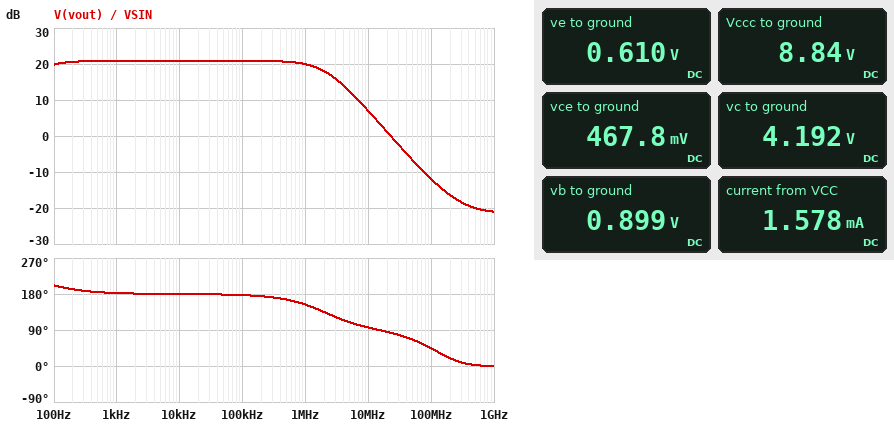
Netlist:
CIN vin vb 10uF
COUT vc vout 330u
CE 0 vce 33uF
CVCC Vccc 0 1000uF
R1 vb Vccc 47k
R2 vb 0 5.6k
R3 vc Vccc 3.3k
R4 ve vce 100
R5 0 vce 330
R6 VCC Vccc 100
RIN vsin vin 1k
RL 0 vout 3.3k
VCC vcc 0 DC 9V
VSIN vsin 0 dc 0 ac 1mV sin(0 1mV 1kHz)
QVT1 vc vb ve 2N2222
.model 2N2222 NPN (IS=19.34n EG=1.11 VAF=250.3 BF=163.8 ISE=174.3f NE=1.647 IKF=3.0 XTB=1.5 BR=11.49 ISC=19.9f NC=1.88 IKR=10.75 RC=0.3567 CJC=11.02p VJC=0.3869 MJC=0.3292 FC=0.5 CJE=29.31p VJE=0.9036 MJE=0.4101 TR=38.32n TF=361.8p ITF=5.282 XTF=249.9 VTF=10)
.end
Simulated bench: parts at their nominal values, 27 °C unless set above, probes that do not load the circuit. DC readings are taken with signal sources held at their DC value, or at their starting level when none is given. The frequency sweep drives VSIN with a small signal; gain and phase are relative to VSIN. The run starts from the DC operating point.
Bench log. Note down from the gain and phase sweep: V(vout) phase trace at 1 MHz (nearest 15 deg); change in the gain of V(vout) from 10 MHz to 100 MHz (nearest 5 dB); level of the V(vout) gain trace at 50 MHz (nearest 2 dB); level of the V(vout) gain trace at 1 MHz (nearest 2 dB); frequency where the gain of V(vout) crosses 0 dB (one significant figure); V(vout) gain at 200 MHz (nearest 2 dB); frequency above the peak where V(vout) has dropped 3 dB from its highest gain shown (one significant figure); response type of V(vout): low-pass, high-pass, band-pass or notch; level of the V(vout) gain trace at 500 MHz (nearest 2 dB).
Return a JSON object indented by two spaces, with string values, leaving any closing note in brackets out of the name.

{
  "V(vout) phase trace at 1 MHz": "150 deg",
  "change in the gain of V(vout) from 10 MHz to 100 MHz": "-20 dB",
  "level of the V(vout) gain trace at 50 MHz": "-6 dB",
  "level of the V(vout) gain trace at 1 MHz": "20 dB",
  "frequency where the gain of V(vout) crosses 0 dB": "20 MHz",
  "V(vout) gain at 200 MHz": "-16 dB",
  "frequency above the peak where V(vout) has dropped 3 dB from its highest gain shown": "2 MHz",
  "response type of V(vout): low-pass, high-pass, band-pass or notch": "low-pass",
  "level of the V(vout) gain trace at 500 MHz": "-20 dB"
}
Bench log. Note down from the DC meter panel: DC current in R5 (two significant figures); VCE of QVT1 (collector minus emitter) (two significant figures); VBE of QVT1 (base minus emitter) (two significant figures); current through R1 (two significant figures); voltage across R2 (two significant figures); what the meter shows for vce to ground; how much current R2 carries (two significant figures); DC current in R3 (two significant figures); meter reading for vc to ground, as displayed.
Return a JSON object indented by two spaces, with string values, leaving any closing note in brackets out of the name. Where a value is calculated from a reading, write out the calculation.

{
  "DC current in R5": "(467.8 mV) / 330 Ω = 1.4 mA",
  "VCE of QVT1 (collector minus emitter)": "4.192 V - 610 mV = 3.6 V",
  "VBE of QVT1 (base minus emitter)": "899 mV - 610 mV = 290 mV",
  "current through R1": "(8.84 V - 899 mV) / 47 kΩ = 170 µA",
  "voltage across R2": "899 mV = 900 mV",
  "what the meter shows for vce to ground": "467.8 mV",
  "how much current R2 carries": "(899 mV) / 5.6 kΩ = 160 µA",
  "DC current in R3": "(8.84 V - 4.192 V) / 3.3 kΩ = 1.4 mA",
  "meter reading for vc to ground, as displayed": "4.192 V"
}
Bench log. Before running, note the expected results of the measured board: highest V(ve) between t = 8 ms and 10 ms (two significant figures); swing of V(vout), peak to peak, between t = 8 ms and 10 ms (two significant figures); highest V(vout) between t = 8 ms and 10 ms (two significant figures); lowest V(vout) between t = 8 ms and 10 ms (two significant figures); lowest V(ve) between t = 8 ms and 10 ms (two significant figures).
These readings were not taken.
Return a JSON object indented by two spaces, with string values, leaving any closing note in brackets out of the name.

{
  "highest V(ve) between t = 8 ms and 10 ms": "610 mV",
  "swing of V(vout), peak to peak, between t = 8 ms and 10 ms": "22 mV",
  "highest V(vout) between t = 8 ms and 10 ms": "11 mV",
  "lowest V(vout) between t = 8 ms and 10 ms": "-11 mV",
  "lowest V(ve) between t = 8 ms and 10 ms": "610 mV"
}
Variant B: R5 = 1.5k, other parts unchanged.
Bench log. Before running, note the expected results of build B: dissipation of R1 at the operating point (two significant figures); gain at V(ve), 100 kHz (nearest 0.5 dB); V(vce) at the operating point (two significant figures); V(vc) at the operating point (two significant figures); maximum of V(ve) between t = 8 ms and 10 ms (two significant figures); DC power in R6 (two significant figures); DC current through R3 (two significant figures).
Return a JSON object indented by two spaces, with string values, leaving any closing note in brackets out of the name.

{
  "dissipation of R1 at the operating point": "1.4 mW",
  "gain at V(ve), 100 kHz": "-6.0 dB",
  "V(vce) at the operating point": "640 mV",
  "V(vc) at the operating point": "7.5 V",
  "maximum of V(ve) between t = 8 ms and 10 ms": "680 mV",
  "DC power in R6": "35 µW",
  "DC current through R3": "420 µA"
}
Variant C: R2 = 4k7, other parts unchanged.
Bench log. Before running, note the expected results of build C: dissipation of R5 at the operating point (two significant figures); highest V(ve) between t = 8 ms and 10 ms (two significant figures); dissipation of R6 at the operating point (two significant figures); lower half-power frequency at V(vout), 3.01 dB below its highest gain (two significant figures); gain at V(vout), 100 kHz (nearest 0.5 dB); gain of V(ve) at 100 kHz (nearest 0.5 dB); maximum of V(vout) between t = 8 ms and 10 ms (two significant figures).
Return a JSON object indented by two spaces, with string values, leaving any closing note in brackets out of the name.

{
  "dissipation of R5 at the operating point": "430 µW",
  "highest V(ve) between t = 8 ms and 10 ms": "490 mV",
  "dissipation of R6 at the operating point": "170 µW",
  "lower half-power frequency at V(vout), 3.01 dB below its highest gain": "49 Hz",
  "gain at V(vout), 100 kHz": "20.5 dB",
  "gain of V(ve) at 100 kHz": "-4.0 dB",
  "maximum of V(vout) between t = 8 ms and 10 ms": "10 mV"
}
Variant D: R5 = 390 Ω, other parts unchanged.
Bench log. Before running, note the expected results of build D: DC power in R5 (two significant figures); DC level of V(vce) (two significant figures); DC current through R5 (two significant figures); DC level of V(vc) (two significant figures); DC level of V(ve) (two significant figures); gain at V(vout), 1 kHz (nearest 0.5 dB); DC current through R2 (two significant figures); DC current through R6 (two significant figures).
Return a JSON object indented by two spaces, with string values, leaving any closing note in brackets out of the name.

{
  "DC power in R5": "620 µW",
  "DC level of V(vce)": "490 mV",
  "DC current through R5": "1.3 mA",
  "DC level of V(vc)": "4.7 V",
  "DC level of V(ve)": "620 mV",
  "gain at V(vout), 1 kHz": "20.5 dB",
  "DC current through R2": "160 µA",
  "DC current through R6": "1.4 mA"
}
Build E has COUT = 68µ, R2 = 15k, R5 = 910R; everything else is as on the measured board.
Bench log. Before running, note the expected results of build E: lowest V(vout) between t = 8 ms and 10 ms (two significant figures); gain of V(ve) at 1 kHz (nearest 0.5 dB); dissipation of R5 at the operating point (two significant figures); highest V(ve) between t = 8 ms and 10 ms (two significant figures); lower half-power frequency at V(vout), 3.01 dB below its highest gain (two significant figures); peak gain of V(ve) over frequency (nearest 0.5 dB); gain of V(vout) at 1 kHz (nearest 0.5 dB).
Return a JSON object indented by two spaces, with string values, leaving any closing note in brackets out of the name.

{
  "lowest V(vout) between t = 8 ms and 10 ms": "-12 mV",
  "gain of V(ve) at 1 kHz": "-2.5 dB",
  "dissipation of R5 at the operating point": "2.6 mW",
  "highest V(ve) between t = 8 ms and 10 ms": "1.7 V",
  "lower half-power frequency at V(vout), 3.01 dB below its highest gain": "45 Hz",
  "peak gain of V(ve) over frequency": "-1.0 dB",
  "gain of V(vout) at 1 kHz": "22.0 dB"
}
